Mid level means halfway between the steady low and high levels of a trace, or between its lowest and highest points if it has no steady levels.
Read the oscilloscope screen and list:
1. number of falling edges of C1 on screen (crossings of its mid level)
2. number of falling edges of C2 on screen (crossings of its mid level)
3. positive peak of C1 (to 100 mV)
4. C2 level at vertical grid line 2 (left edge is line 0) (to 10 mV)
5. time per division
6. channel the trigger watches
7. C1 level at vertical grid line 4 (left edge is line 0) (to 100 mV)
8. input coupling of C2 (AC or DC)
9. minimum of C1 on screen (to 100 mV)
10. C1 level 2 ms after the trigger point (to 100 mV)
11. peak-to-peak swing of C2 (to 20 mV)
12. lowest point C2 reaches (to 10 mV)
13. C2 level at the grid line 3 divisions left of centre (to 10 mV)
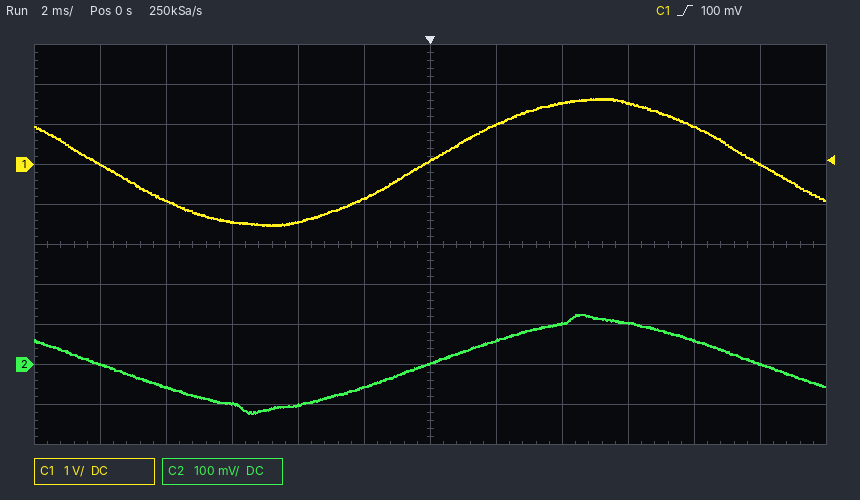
2
2
1.6 V
-60 mV
2 ms
C1
-1.4 V
DC
-1.5 V
1.0 V
240 mV
-120 mV
-100 mV
